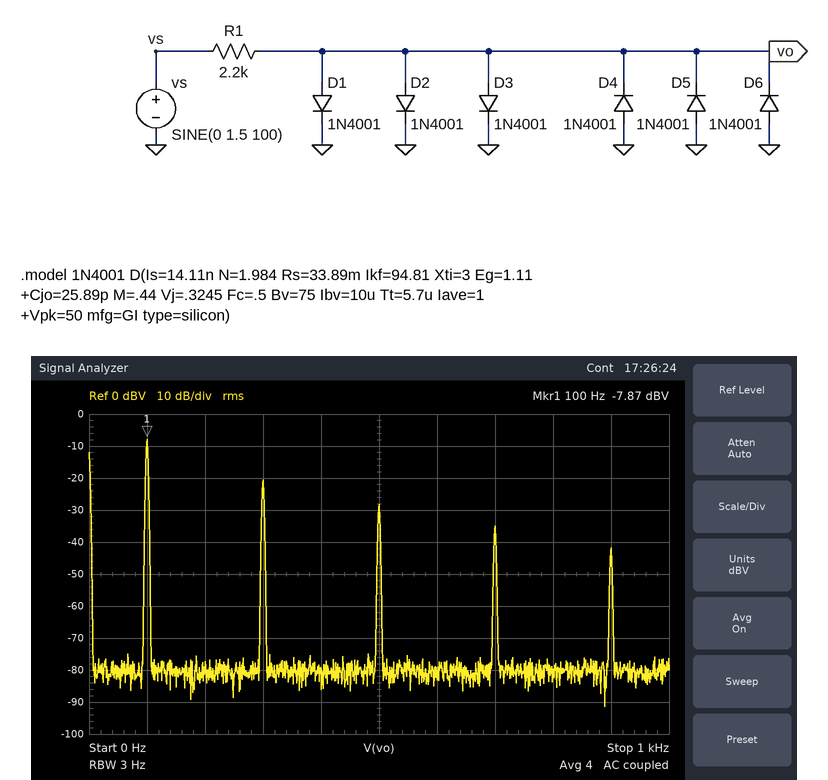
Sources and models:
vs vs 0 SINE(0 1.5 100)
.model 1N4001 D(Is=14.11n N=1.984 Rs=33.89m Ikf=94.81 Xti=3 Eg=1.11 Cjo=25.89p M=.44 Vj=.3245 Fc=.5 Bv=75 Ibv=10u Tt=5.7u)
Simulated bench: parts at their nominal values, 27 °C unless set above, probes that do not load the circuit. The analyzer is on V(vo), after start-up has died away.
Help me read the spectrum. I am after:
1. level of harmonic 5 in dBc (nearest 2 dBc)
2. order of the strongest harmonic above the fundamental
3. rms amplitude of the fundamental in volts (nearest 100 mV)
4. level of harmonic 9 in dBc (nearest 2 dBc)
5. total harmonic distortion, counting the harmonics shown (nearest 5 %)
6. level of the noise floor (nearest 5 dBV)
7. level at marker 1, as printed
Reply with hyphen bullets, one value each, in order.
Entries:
- -20 dBc
- 3
- 400 mV
- -34 dBc
- 25 %
- -80 dBV
- -7.87 dBV
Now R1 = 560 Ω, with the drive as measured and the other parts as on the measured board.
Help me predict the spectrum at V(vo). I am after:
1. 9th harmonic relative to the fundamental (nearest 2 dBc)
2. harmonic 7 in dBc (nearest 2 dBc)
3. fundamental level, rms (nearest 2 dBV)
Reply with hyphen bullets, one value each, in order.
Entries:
- -38 dBc
- -30 dBc
- -6 dBV
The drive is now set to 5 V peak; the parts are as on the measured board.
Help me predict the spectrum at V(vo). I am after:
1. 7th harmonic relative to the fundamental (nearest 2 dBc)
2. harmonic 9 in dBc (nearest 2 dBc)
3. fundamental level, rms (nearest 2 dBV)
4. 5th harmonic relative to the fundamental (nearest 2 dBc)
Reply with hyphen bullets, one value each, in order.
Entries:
- -20 dBc
- -24 dBc
- -6 dBV
- -16 dBc
